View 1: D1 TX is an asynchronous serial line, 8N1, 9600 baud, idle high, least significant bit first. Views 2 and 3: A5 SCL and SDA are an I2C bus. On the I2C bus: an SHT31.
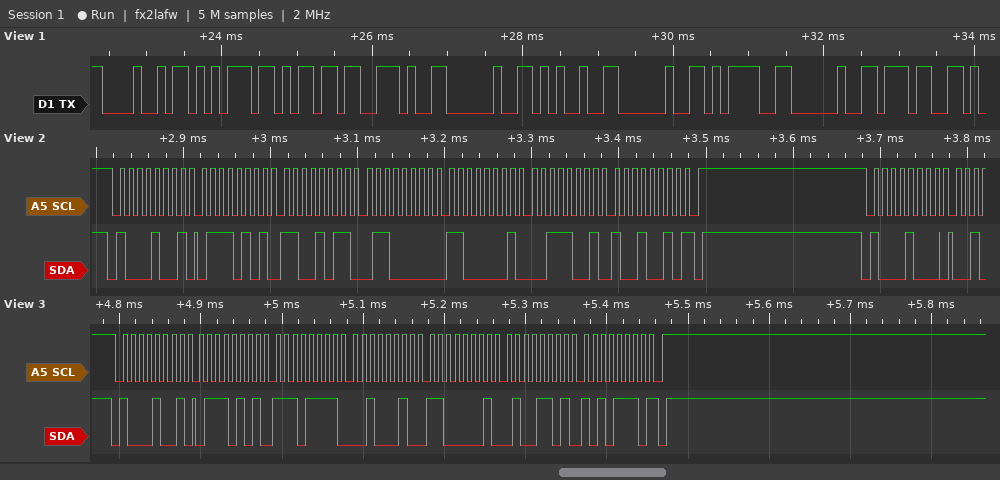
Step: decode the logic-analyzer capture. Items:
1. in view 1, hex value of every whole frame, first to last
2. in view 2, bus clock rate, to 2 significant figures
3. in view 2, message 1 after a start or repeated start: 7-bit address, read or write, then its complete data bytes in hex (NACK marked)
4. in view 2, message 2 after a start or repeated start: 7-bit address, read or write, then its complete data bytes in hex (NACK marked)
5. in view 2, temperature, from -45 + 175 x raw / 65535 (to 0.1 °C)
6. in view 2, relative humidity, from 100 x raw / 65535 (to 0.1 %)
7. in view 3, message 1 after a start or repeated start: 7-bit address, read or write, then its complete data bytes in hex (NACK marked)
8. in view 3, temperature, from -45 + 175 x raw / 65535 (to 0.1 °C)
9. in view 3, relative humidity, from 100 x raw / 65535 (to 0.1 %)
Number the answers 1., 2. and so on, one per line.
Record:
1. 48 75 6D 2E 20 25 20 3D 20 37
2. 100 kHz
3. 0x44 read: 75 CB 60 C1 39 92 NACK
4. 0x44 write
5. 35.5 °C
6. 75.5 %
7. 0x44 read: 75 EF 22 C1 4D AE NACK
8. 35.6 °C
9. 75.5 %
